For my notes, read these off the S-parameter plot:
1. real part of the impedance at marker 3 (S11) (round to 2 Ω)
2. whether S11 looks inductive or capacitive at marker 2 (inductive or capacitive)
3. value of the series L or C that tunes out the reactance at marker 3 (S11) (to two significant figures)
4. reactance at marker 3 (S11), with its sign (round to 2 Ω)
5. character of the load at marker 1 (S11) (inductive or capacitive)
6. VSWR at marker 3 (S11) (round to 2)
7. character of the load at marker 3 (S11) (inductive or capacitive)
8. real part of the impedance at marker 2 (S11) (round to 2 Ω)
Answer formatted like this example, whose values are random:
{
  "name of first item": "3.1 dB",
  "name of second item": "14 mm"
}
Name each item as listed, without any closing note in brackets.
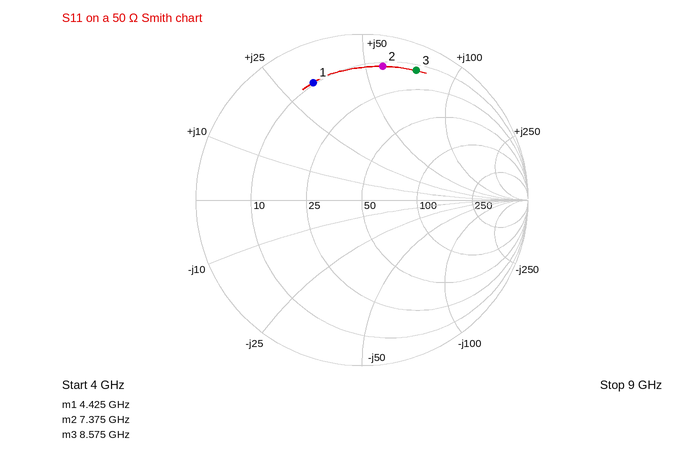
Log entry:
{
  "real part of the impedance at marker 3 (S11)": "14 Ω",
  "whether S11 looks inductive or capacitive at marker 2": "inductive",
  "value of the series L or C that tunes out the reactance at marker 3 (S11)": "250 fF",
  "reactance at marker 3 (S11), with its sign": "+74 Ω",
  "character of the load at marker 1 (S11)": "inductive",
  "VSWR at marker 3 (S11)": "12",
  "character of the load at marker 3 (S11)": "inductive",
  "real part of the impedance at marker 2 (S11)": "12 Ω"
}
